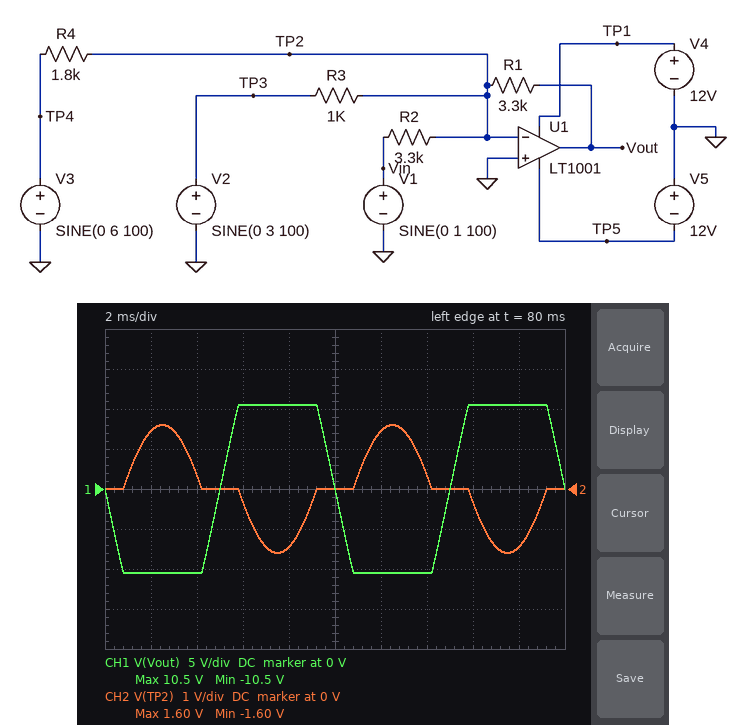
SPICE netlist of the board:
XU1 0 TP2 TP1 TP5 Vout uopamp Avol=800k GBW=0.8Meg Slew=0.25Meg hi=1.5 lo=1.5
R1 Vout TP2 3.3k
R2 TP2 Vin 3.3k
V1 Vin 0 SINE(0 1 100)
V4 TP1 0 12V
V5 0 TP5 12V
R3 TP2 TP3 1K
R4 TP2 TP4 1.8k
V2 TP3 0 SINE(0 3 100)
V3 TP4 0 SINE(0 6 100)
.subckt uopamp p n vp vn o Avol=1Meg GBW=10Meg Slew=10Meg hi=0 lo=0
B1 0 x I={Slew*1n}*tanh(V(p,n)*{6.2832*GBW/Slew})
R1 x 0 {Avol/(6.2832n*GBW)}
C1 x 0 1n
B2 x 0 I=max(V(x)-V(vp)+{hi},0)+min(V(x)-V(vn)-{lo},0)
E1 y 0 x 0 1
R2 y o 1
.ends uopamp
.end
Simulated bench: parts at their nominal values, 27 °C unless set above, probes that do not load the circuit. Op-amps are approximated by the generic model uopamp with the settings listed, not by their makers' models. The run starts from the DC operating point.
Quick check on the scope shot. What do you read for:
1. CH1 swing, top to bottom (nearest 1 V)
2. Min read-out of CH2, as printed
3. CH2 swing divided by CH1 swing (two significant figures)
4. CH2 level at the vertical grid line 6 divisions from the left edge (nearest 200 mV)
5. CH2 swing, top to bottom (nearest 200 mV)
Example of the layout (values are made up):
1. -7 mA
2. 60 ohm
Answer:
1. 21 V
2. -1.60 V
3. 0.15
4. 1.4 V
5. 3.2 V
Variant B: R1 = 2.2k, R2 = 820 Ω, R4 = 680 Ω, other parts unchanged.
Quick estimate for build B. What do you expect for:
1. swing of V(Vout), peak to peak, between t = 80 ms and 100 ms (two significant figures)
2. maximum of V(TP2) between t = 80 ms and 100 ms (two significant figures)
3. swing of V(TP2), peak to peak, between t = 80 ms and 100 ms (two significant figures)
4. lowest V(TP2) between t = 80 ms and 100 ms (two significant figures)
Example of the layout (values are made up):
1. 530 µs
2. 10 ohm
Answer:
1. 21 V
2. 2.0 V
3. 4.0 V
4. -2.0 V
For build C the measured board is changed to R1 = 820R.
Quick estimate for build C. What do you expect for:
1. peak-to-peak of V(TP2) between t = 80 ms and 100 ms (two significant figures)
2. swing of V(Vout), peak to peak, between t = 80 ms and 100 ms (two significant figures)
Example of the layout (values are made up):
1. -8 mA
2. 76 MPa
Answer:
1. 1.4 mV
2. 11 V
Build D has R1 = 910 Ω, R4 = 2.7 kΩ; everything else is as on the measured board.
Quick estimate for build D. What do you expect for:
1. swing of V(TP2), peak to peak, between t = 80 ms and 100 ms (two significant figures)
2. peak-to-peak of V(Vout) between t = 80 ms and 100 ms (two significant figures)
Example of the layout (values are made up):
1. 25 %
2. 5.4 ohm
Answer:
1. 1.3 mV
2. 10 V
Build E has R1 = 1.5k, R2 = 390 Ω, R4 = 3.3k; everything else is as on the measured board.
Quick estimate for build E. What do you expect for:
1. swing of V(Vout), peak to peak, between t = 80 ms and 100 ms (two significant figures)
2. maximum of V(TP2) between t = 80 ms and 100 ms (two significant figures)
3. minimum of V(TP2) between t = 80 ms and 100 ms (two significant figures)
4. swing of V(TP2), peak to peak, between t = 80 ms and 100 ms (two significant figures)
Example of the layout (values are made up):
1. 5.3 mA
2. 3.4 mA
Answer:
1. 21 V
2. 85 mV
3. -85 mV
4. 170 mV
